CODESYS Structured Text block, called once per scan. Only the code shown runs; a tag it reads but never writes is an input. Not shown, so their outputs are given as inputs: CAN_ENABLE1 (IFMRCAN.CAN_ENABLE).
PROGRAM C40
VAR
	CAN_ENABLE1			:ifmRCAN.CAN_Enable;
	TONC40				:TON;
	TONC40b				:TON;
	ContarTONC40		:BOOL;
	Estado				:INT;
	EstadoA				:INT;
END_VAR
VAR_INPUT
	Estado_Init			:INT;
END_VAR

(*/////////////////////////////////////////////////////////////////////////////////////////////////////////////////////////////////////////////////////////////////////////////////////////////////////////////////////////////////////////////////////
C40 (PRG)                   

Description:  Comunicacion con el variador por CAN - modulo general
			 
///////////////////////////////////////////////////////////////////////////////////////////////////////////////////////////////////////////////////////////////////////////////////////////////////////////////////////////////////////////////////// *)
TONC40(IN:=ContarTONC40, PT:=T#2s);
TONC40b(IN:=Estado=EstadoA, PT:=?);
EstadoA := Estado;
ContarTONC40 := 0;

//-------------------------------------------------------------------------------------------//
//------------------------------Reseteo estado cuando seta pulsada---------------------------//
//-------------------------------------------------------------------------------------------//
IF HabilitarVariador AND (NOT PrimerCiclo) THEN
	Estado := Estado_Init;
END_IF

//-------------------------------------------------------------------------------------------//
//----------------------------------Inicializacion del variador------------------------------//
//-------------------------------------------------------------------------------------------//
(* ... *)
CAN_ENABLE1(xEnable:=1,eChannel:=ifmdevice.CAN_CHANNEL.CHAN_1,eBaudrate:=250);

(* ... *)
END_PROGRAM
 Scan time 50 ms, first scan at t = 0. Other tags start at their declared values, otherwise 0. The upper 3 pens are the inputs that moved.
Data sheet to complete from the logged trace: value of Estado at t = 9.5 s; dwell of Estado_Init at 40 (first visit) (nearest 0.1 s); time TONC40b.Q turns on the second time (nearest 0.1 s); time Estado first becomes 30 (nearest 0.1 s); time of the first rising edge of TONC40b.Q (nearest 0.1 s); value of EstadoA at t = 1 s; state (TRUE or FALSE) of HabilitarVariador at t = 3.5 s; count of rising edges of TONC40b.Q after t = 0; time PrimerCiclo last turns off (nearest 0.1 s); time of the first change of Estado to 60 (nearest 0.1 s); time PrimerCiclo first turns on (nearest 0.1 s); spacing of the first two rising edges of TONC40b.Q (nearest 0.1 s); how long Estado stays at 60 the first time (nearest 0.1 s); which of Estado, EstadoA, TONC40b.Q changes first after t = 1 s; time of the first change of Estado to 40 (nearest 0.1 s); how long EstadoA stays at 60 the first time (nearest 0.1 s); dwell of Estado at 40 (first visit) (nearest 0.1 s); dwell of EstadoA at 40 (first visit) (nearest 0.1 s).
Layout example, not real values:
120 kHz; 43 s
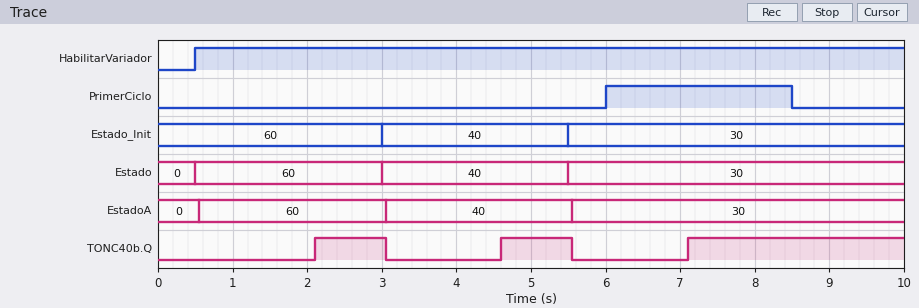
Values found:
30; 2.5 s; 4.6 s; 5.5 s; 2.1 s; 60; TRUE; 3; 8.5 s; 0.5 s; 6.0 s; 2.5 s; 2.5 s; TONC40b.Q; 3.0 s; 2.5 s; 2.5 s; 2.5 s
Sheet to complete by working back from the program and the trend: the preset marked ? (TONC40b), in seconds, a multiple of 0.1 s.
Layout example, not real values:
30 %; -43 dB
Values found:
1.5 s
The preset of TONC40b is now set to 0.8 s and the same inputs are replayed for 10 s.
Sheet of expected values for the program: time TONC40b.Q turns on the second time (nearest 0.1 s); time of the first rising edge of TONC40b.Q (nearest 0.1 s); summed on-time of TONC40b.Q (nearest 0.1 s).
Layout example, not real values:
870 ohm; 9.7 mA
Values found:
3.9 s; 1.4 s; 6.9 s
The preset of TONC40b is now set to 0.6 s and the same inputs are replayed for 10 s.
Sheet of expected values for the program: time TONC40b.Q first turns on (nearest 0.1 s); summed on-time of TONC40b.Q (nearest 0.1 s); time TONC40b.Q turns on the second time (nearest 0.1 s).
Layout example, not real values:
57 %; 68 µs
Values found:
1.2 s; 7.5 s; 3.7 s
